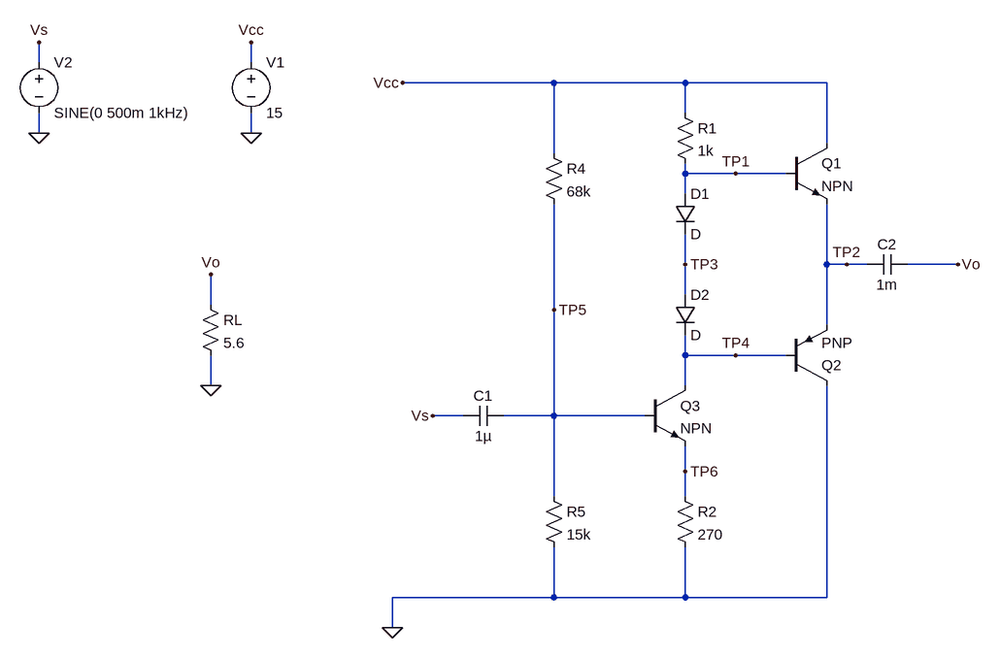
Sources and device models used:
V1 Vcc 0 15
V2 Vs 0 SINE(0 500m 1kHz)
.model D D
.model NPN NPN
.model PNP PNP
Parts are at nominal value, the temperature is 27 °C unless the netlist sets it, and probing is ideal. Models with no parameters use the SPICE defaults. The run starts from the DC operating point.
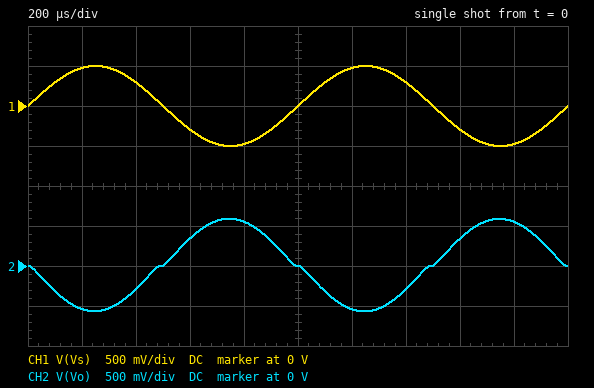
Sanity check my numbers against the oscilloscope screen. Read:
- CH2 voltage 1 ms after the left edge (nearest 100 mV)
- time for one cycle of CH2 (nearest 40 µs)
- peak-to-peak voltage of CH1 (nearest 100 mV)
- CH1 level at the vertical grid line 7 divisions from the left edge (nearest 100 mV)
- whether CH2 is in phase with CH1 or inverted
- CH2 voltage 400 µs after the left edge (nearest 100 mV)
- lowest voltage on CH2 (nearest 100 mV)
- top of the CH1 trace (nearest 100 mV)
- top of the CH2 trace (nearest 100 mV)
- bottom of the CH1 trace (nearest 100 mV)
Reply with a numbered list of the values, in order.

1. 0 V
2. 1.00 ms
3. 1.0 V
4. 300 mV
5. inverted
6. -300 mV
7. -600 mV
8. 500 mV
9. 600 mV
10. -500 mV
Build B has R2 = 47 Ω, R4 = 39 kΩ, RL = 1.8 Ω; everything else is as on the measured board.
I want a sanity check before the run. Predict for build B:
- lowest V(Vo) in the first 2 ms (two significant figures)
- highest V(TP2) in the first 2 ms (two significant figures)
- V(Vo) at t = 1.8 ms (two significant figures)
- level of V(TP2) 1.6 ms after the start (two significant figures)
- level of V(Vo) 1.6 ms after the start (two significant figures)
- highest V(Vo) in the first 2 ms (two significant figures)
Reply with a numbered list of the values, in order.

1. -300 mV
2. 4.1 V
3. 1.8 V
4. 3.8 V
5. 1.7 V
6. 1.9 V
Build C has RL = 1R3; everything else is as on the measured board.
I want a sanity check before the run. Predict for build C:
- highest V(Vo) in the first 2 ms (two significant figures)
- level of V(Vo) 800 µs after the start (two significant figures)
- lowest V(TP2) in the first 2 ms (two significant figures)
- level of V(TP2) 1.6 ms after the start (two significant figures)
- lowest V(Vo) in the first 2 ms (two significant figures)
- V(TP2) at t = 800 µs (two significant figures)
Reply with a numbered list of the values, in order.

1. 190 mV
2. 180 mV
3. 9.3 V
4. 9.6 V
5. -180 mV
6. 9.7 V
